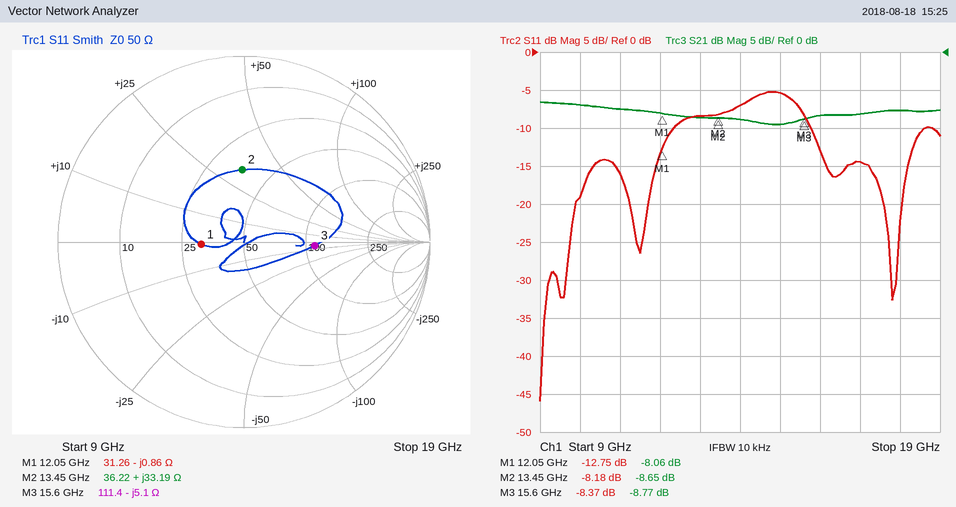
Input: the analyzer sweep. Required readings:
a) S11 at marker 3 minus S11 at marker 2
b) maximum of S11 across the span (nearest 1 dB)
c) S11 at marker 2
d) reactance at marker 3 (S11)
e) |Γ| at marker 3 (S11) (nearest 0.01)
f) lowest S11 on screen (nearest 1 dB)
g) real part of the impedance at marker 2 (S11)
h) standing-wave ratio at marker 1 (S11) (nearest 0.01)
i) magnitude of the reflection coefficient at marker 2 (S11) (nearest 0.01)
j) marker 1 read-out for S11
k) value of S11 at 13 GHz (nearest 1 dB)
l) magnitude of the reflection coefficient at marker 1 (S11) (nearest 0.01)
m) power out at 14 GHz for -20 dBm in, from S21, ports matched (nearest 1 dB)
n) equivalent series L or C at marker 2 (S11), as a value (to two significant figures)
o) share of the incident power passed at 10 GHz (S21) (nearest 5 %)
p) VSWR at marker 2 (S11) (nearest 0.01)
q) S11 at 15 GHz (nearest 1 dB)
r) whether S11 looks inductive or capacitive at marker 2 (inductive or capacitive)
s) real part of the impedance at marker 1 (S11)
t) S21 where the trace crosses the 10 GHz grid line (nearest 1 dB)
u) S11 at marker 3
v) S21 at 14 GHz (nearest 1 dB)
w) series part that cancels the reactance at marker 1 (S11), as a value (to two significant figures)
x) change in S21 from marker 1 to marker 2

-0.19 dB
-5 dB
-8.18 dB
-5.1 Ω
0.38
-46 dB
36.22 Ω
1.60
0.39
-12.75 dB
-8 dB
0.23
-29 dBm
390 pH
20 %
2.28
-5 dB
inductive
31.26 Ω
-7 dB
-8.37 dB
-9 dB
11 pH
-0.59 dB
